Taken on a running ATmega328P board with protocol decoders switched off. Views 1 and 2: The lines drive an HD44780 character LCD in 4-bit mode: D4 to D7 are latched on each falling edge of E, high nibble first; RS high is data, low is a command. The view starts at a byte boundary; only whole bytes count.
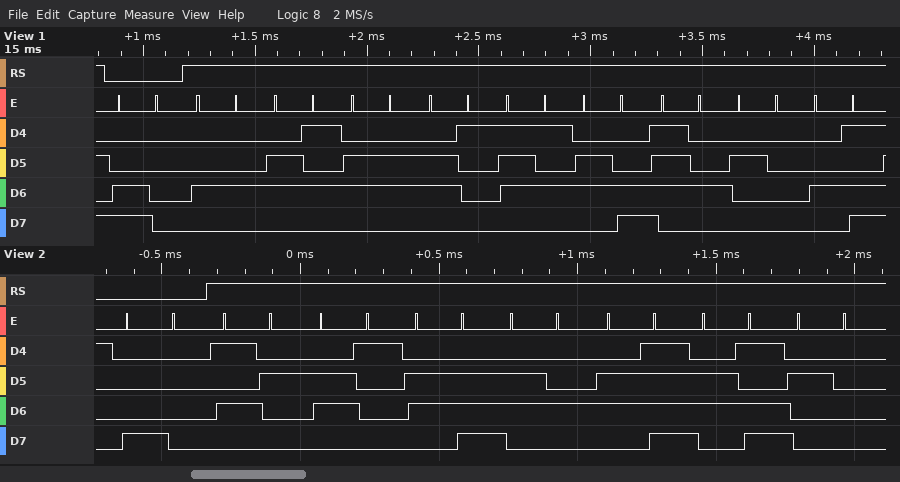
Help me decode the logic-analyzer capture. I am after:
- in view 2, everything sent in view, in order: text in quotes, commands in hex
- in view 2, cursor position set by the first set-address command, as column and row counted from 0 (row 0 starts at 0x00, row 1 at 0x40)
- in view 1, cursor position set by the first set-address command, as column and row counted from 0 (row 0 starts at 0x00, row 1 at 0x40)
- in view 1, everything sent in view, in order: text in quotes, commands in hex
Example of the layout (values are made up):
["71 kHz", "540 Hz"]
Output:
["0x80 \"Random \"", "column 0, row 0", "column 0, row 1", "0xC0 \"Default M\""]
